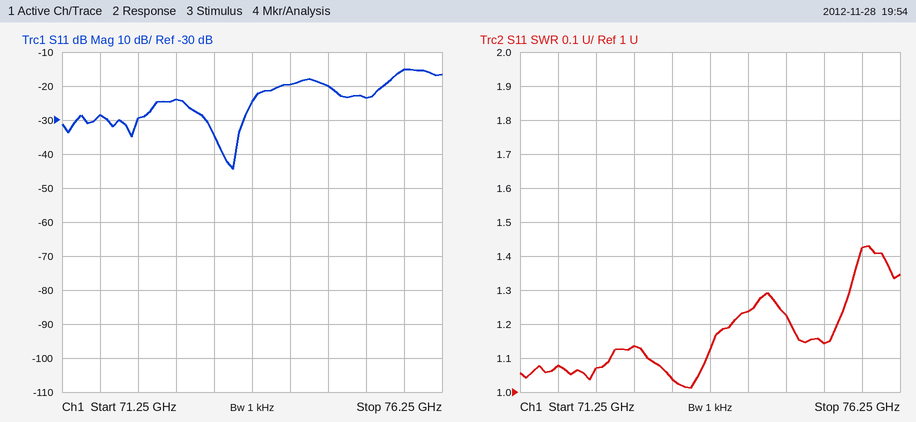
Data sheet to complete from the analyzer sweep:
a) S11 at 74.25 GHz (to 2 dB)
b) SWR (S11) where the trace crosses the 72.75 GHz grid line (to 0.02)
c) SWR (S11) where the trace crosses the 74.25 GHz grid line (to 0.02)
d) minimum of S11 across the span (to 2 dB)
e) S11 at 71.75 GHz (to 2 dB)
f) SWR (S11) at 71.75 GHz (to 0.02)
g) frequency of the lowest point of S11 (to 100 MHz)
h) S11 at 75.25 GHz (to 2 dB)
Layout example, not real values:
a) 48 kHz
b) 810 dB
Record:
a) -20 dB
b) 1.14
c) 1.24
d) -44 dB
e) -28 dB
f) 1.08
g) 73.5 GHz
h) -24 dB
